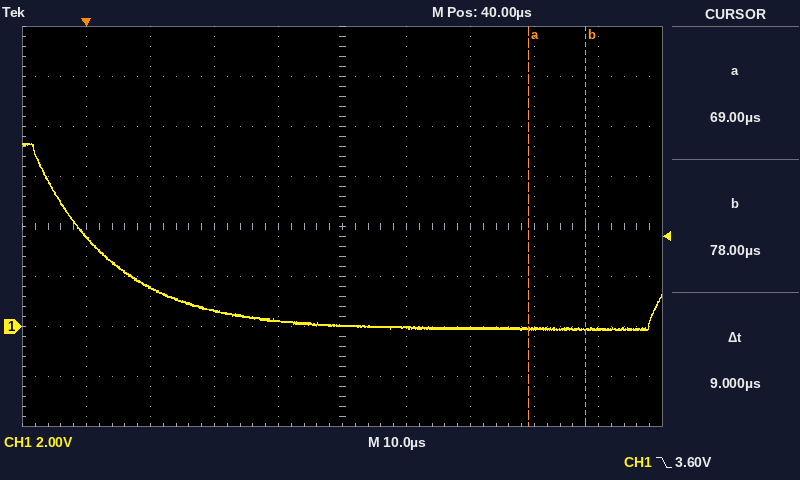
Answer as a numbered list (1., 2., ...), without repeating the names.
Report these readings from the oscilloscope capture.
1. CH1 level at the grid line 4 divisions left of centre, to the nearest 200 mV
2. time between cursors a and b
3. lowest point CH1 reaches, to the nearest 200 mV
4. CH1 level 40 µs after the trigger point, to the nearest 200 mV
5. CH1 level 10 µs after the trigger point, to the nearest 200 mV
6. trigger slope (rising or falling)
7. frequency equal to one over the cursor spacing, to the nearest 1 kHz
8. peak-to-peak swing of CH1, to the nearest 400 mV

1. 3.6 V
2. 9 µs
3. -200 mV
4. 0.0 V
5. 1.6 V
6. falling
7. 111 kHz
8. 7.6 V
